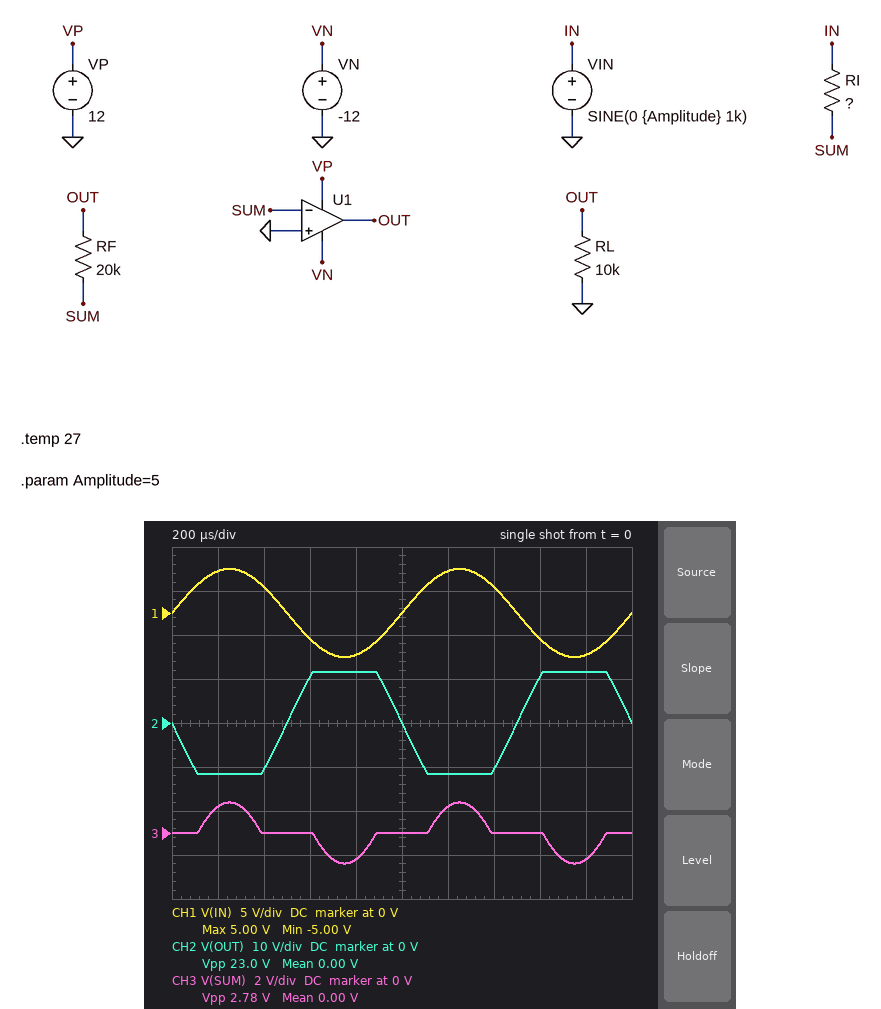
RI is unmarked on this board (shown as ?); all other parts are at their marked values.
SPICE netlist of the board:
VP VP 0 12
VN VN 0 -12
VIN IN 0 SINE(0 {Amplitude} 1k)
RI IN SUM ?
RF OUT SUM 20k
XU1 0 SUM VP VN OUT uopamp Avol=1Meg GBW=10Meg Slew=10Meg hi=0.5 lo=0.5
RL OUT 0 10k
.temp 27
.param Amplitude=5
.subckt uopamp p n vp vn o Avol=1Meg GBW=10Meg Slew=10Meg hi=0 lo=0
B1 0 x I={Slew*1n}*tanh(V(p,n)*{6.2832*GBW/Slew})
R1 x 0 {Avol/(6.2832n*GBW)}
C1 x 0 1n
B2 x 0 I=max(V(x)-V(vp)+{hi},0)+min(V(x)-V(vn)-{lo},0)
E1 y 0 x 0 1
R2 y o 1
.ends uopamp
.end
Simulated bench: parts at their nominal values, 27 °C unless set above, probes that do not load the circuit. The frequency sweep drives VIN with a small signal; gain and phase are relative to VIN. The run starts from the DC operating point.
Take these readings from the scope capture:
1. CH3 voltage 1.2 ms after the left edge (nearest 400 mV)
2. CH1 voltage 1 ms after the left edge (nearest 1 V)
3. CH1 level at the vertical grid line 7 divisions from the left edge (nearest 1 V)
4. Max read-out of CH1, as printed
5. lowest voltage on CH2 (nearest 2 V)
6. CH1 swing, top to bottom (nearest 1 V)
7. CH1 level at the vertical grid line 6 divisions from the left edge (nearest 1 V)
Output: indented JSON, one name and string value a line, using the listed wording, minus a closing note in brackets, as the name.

{
  "CH3 voltage 1.2 ms after the left edge": "1.2 V",
  "CH1 voltage 1 ms after the left edge": "0 V",
  "CH1 level at the vertical grid line 7 divisions from the left edge": "3 V",
  "Max read-out of CH1, as printed": "5.00 V",
  "lowest voltage on CH2": "-12 V",
  "CH1 swing, top to bottom": "10 V",
  "CH1 level at the vertical grid line 6 divisions from the left edge": "5 V"
}
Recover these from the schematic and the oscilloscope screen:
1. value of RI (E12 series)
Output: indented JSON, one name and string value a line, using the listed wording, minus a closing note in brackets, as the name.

{
  "value of RI": "5.6 kΩ"
}
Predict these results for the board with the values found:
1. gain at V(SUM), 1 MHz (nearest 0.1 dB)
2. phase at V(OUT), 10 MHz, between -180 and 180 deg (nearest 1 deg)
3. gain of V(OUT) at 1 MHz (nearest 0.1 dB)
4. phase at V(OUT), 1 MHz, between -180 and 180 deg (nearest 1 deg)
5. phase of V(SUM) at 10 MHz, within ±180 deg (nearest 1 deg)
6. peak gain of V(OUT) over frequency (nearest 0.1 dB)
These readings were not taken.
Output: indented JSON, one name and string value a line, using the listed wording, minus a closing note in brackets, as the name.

{
  "gain at V(SUM), 1 MHz": "-9.8 dB",
  "phase at V(OUT), 10 MHz, between -180 and 180 deg": "102 deg",
  "gain of V(OUT) at 1 MHz": "10.2 dB",
  "phase at V(OUT), 1 MHz, between -180 and 180 deg": "155 deg",
  "phase of V(SUM) at 10 MHz, within ±180 deg": "12 deg",
  "peak gain of V(OUT) over frequency": "11.1 dB"
}
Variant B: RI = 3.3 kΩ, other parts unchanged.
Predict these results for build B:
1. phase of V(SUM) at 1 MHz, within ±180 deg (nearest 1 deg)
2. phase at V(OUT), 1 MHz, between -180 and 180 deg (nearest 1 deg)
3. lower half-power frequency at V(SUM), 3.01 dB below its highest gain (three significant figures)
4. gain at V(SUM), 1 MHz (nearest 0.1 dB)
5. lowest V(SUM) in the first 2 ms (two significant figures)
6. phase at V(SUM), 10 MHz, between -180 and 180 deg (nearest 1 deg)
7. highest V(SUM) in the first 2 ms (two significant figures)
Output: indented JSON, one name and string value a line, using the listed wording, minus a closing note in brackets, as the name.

{
  "phase of V(SUM) at 1 MHz, within ±180 deg": "55 deg",
  "phase at V(OUT), 1 MHz, between -180 and 180 deg": "145 deg",
  "lower half-power frequency at V(SUM), 3.01 dB below its highest gain": "1.42 MHz",
  "gain at V(SUM), 1 MHz": "-6.1 dB",
  "lowest V(SUM) in the first 2 ms": "-2.7 V",
  "phase at V(SUM), 10 MHz, between -180 and 180 deg": "8 deg",
  "highest V(SUM) in the first 2 ms": "2.7 V"
}
